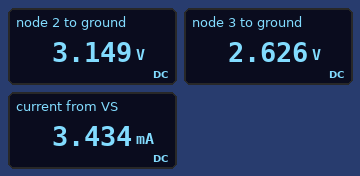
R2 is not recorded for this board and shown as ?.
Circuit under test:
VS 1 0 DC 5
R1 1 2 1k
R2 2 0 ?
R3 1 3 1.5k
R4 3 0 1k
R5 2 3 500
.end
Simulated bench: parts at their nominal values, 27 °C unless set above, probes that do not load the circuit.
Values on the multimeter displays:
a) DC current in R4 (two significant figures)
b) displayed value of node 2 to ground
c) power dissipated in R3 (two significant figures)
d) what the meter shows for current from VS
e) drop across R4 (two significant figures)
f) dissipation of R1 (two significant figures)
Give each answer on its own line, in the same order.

2.6 mA
3.149 V
3.8 mW
3.434 mA
2.6 V
3.4 mW
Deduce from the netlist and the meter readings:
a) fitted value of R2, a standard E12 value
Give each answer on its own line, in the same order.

3.9 kΩ
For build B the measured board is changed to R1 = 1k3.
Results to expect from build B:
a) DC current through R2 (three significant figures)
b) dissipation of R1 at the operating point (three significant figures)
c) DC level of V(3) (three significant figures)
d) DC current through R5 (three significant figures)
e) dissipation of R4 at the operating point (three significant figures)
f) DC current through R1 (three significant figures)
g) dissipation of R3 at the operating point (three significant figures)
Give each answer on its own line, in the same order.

751 µA
3.30 mW
2.51 V
843 µA
6.28 mW
1.59 mA
4.15 mW
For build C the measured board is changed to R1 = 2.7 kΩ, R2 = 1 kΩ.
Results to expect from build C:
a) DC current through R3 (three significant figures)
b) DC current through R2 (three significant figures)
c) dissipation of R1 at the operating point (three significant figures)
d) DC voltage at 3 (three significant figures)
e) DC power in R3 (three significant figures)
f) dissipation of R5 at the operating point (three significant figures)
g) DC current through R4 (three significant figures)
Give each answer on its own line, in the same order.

2.14 mA
1.61 mA
4.26 mW
1.79 V
6.88 mW
62.8 µW
1.79 mA
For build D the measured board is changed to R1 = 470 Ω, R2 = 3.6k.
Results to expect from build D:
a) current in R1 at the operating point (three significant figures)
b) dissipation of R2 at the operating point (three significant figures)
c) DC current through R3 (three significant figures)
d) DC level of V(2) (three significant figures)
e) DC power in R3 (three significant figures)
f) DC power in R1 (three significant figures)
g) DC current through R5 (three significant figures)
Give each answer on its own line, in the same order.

2.64 mA
3.92 mW
1.36 mA
3.76 V
2.78 mW
3.28 mW
1.60 mA
